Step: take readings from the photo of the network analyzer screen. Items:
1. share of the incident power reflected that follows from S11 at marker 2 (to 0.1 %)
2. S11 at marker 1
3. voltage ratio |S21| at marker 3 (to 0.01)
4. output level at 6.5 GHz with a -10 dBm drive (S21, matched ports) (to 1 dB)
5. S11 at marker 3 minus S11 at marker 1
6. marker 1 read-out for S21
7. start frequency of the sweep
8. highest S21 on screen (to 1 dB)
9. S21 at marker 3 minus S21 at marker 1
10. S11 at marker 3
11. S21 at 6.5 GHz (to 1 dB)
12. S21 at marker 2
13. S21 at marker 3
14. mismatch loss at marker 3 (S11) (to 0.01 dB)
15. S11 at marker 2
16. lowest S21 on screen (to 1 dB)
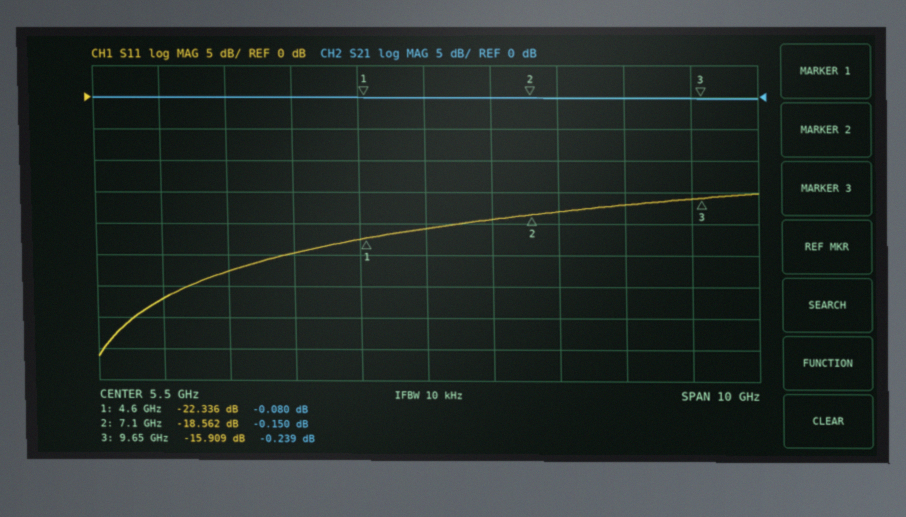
1.4 %
-22.336 dB
0.97
-10 dBm
6.427 dB
-0.080 dB
500 MHz
0 dB
-0.159 dB
-15.909 dB
0 dB
-0.150 dB
-0.239 dB
0.11 dB
-18.562 dB
0 dB
